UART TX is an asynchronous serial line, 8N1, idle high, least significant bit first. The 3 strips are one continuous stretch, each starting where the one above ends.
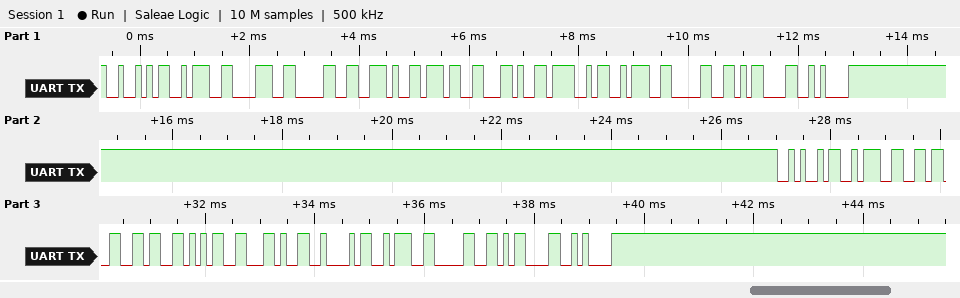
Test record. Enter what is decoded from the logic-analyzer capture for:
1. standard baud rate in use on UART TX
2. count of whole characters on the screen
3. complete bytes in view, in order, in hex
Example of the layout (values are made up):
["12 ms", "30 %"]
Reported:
["9600 baud", "23", "52 3A 38 30 2E 37 2C 4F 3A 30 0D 0A 4A 3A 36 36 35 2C 42 3A 30 0D 0A"]
